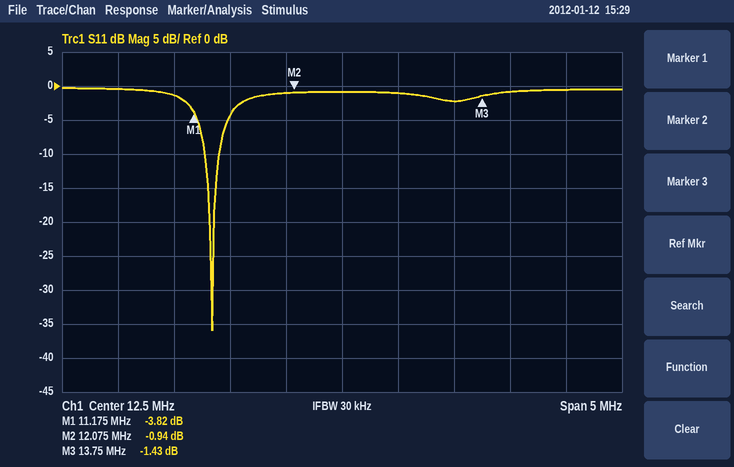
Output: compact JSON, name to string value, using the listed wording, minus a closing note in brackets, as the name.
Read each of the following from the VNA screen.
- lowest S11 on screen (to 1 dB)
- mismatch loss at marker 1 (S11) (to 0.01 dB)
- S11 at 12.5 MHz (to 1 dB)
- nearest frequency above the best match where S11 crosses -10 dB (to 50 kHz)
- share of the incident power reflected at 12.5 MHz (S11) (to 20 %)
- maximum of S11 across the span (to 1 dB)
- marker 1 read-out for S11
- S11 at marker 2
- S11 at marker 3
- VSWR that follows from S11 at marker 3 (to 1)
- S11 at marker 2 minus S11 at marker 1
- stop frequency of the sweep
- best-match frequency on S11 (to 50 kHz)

{"lowest S11 on screen": "-36 dB", "mismatch loss at marker 1 (S11)": "2.33 dB", "S11 at 12.5 MHz": "-1 dB", "nearest frequency above the best match where S11 crosses -10 dB": "11.40 MHz", "share of the incident power reflected at 12.5 MHz (S11)": "80 %", "maximum of S11 across the span": "0 dB", "marker 1 read-out for S11": "-3.82 dB", "S11 at marker 2": "-0.94 dB", "S11 at marker 3": "-1.43 dB", "VSWR that follows from S11 at marker 3": "12", "S11 at marker 2 minus S11 at marker 1": "2.88 dB", "stop frequency of the sweep": "15 MHz", "best-match frequency on S11": "11.35 MHz"}
